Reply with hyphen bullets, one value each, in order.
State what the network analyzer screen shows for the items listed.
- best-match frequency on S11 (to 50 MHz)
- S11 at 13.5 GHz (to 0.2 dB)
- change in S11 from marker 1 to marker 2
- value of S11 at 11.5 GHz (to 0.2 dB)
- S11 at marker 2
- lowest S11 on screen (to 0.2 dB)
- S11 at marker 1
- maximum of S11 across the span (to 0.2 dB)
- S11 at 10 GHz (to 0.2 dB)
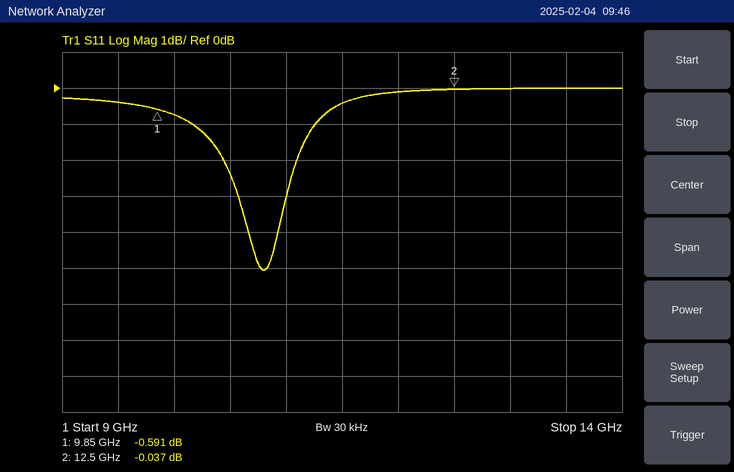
- 10.80 GHz
- 0.0 dB
- 0.554 dB
- -0.4 dB
- -0.037 dB
- -5.0 dB
- -0.591 dB
- 0.0 dB
- -0.8 dB
